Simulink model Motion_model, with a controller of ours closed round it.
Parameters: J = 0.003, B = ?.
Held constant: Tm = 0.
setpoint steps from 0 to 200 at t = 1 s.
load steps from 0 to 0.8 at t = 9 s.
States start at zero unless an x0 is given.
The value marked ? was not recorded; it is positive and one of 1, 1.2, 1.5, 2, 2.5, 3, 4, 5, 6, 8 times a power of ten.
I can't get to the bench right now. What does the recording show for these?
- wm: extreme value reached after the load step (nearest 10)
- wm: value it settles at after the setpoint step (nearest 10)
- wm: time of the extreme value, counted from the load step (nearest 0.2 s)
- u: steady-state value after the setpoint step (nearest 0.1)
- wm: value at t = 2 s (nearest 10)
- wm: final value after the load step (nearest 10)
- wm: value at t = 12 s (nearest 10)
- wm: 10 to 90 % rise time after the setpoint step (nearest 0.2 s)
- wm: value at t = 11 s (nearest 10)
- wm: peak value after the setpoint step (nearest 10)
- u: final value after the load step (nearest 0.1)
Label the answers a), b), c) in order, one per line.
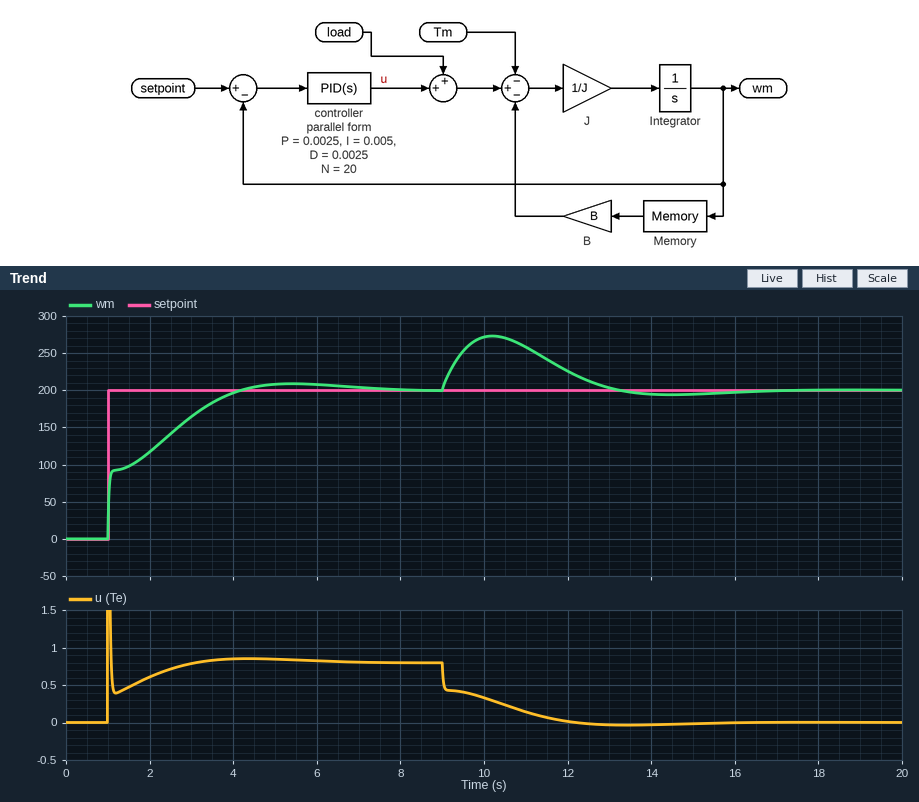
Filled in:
a) 270
b) 200
c) 1.2 s
d) 0.8
e) 120
f) 200
g) 230
h) 2.4 s
i) 260
j) 210
k) 0.0
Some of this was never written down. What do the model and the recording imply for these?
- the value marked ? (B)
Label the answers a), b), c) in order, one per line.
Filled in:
a) 0.004
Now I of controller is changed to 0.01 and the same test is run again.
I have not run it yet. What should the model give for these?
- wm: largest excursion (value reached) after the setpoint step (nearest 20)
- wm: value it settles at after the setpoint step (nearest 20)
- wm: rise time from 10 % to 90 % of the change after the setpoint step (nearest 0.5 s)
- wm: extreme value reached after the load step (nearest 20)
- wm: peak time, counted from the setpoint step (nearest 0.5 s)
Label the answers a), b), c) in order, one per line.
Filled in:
a) 220
b) 200
c) 1.5 s
d) 260
e) 2.5 s
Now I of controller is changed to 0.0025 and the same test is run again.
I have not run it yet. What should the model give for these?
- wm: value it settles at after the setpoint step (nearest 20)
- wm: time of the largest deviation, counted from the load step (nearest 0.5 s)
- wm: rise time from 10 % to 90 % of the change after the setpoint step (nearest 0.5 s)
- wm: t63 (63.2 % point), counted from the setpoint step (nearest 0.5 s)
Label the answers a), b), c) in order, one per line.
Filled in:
a) 200
b) 1.5 s
c) 4.5 s
d) 2.0 s
